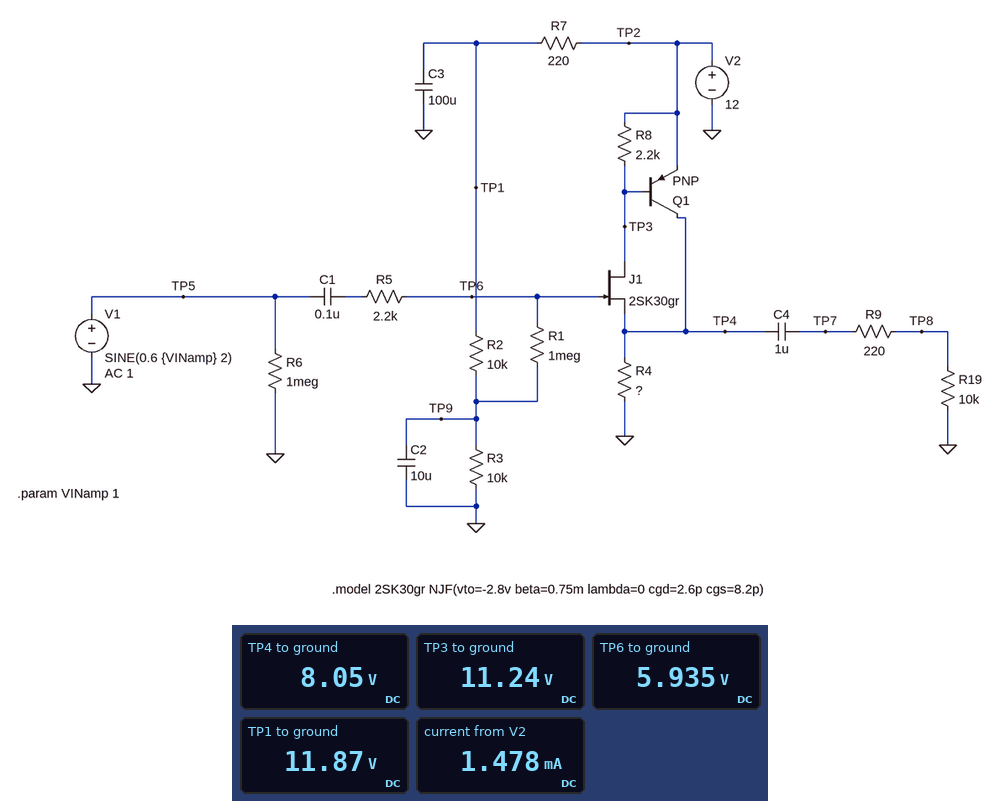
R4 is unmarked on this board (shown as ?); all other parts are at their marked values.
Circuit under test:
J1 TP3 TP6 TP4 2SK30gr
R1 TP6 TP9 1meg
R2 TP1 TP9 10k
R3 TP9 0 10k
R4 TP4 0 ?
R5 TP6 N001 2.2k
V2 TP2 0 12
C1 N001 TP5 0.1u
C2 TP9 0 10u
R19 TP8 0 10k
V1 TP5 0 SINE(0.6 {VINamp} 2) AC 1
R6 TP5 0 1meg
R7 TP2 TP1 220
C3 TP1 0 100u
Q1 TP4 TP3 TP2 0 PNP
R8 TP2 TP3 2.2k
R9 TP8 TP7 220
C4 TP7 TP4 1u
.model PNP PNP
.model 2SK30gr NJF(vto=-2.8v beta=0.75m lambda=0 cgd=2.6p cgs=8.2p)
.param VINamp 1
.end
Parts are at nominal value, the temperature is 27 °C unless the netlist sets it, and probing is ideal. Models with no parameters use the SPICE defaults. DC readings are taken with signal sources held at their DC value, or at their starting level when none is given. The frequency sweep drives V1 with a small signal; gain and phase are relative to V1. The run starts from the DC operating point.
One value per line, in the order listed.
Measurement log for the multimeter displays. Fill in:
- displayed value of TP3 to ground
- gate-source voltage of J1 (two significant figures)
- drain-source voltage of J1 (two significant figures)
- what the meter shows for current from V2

11.24 V
-2.1 V
3.2 V
1.478 mA
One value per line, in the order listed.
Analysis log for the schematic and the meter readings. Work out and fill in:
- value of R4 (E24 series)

9.1 kΩ
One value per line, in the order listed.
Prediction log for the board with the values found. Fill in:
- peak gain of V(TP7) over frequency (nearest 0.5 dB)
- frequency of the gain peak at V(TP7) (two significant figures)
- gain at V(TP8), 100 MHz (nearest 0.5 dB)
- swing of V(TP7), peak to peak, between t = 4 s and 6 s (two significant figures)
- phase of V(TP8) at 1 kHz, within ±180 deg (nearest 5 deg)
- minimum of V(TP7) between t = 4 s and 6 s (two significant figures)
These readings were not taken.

3.0 dB
41 MHz
-11.0 dB
200 mV
0 deg
-99 mV
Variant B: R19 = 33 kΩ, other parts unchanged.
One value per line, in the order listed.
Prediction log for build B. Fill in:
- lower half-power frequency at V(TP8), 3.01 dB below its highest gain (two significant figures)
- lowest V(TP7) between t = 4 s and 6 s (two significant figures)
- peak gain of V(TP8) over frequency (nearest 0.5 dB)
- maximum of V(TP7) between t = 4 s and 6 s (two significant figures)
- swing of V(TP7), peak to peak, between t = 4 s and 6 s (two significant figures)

43 Hz
-300 mV
3.0 dB
300 mV
600 mV
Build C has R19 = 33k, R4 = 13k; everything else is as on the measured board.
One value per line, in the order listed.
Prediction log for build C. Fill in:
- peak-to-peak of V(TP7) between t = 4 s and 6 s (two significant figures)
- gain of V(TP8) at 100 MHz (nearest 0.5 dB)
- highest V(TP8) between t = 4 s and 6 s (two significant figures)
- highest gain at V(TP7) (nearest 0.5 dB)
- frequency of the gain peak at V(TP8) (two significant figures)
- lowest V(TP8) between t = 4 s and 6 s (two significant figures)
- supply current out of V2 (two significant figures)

600 mV
-12.0 dB
300 mV
2.5 dB
39 MHz
-300 mV
1.2 mA
